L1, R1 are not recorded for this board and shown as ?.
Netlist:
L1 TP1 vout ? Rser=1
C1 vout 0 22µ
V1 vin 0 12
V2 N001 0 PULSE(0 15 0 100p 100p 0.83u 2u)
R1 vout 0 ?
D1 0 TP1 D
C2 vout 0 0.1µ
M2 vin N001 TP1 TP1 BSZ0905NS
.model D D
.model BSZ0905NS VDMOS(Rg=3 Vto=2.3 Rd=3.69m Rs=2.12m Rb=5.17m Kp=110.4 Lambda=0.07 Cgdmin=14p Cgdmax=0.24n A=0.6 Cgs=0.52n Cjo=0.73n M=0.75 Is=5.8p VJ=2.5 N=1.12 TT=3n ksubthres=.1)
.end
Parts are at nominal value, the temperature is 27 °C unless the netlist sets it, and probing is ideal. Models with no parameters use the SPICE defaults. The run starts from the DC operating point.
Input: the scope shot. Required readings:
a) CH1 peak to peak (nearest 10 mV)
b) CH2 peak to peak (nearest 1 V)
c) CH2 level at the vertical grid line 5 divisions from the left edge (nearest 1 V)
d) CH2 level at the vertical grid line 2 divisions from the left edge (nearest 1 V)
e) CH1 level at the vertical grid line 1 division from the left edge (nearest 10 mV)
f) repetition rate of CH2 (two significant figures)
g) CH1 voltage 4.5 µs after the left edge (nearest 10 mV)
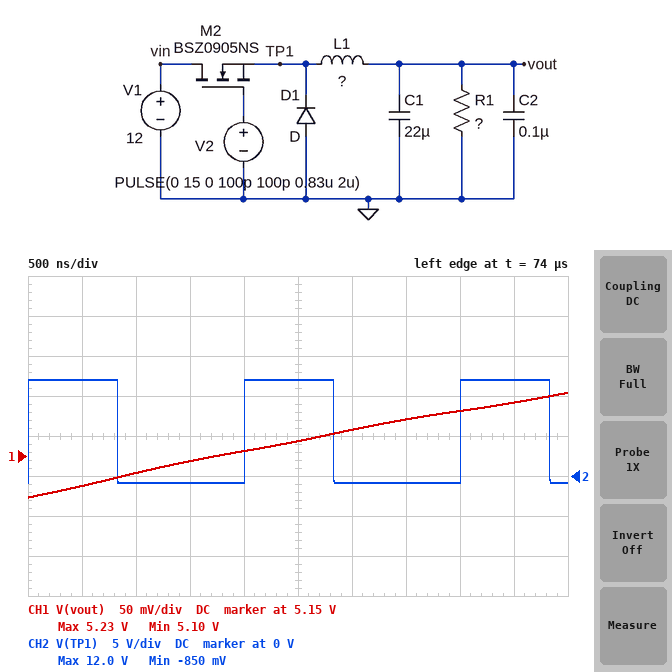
130 mV
13 V
12 V
-1 V
5.11 V
500 kHz
5.22 V
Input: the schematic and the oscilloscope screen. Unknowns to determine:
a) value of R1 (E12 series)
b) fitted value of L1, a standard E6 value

33 Ω
33 µH
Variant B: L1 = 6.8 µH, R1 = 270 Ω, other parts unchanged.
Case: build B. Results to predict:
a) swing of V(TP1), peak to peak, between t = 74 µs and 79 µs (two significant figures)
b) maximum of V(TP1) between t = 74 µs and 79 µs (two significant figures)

14 V
13 V
